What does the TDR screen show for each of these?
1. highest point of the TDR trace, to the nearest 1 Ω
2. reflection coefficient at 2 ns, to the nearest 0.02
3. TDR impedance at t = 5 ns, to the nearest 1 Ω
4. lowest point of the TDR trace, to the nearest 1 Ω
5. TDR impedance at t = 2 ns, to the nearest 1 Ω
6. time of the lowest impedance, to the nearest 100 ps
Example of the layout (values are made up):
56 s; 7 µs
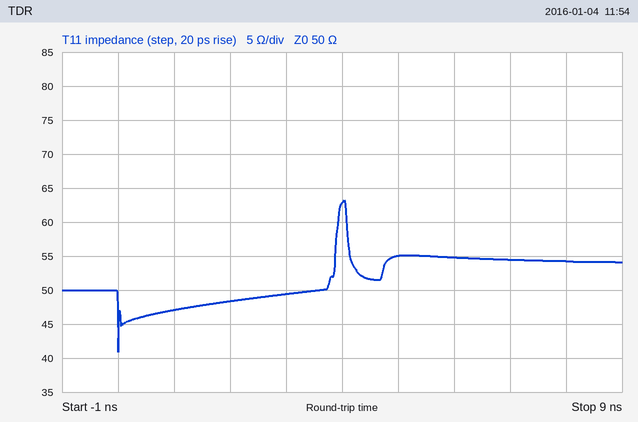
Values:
63 Ω; -0.02; 55 Ω; 41 Ω; 48 Ω; 0.0 ns
